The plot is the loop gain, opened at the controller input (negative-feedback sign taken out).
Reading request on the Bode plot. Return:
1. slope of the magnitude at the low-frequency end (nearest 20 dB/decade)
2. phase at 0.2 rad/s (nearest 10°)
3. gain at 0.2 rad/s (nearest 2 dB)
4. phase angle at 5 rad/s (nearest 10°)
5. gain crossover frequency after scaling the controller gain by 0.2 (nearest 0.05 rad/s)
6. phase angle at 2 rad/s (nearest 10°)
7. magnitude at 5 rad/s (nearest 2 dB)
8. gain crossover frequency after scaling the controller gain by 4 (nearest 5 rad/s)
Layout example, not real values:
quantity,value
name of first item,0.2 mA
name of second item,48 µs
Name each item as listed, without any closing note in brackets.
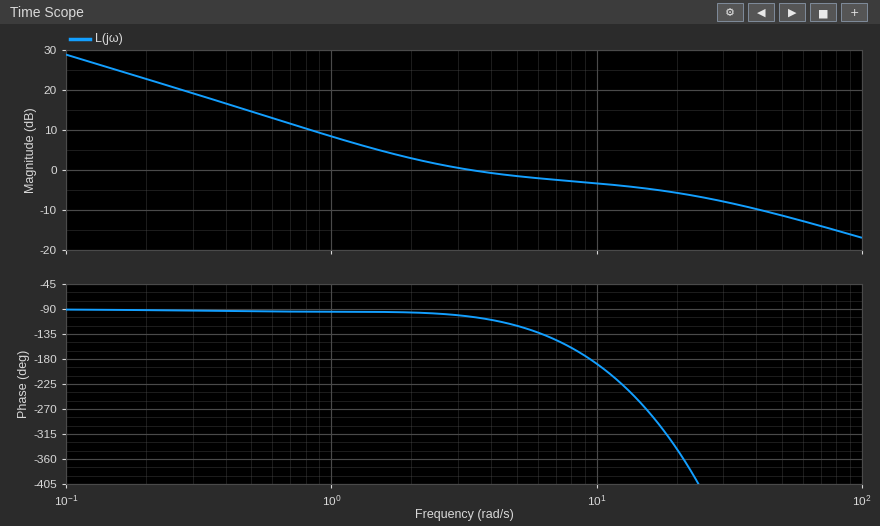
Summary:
quantity,value
slope of the magnitude at the low-frequency end,-20 dB/decade
phase at 0.2 rad/s,-90°
gain at 0.2 rad/s,22 dB
phase angle at 5 rad/s,-120°
gain crossover frequency after scaling the controller gain by 0.2,0.55 rad/s
phase angle at 2 rad/s,-100°
magnitude at 5 rad/s,-2 dB
gain crossover frequency after scaling the controller gain by 4,55 rad/s
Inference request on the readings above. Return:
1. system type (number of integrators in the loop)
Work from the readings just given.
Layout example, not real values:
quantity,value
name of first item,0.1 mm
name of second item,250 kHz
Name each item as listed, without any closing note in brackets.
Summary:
quantity,value
system type,1
